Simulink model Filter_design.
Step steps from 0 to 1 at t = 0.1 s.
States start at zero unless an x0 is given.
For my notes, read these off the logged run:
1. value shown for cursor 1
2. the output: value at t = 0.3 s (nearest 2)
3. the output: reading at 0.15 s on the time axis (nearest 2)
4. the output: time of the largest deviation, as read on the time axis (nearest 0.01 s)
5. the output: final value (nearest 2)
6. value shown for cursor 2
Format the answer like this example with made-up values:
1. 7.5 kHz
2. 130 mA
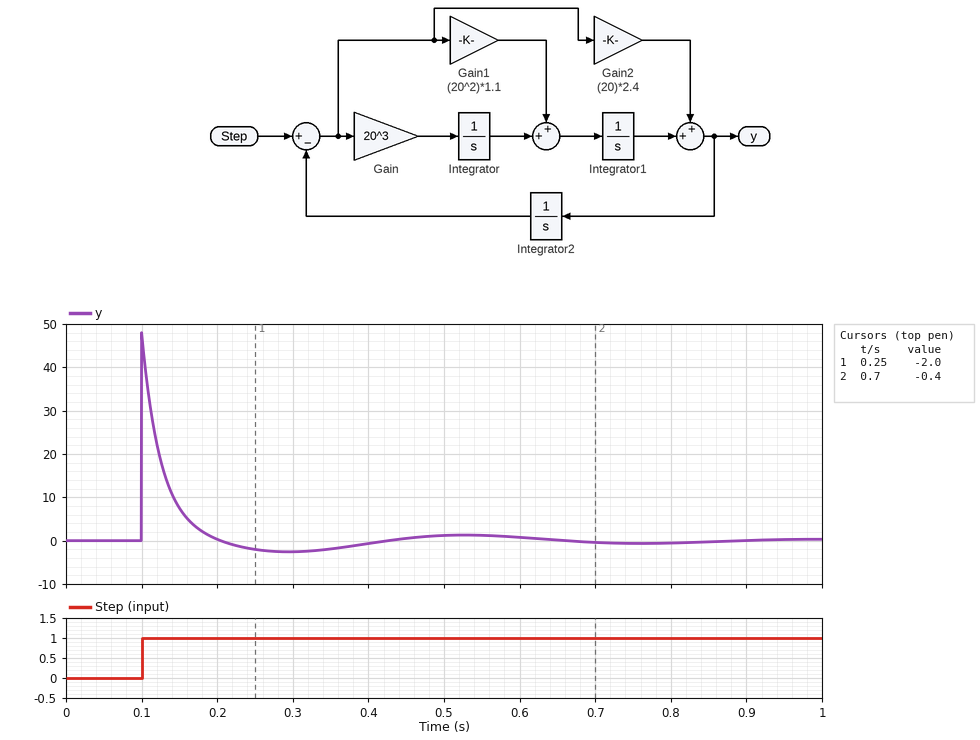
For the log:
1. -2.0
2. -2
3. 8
4. 0.10 s
5. 0
6. -0.4
